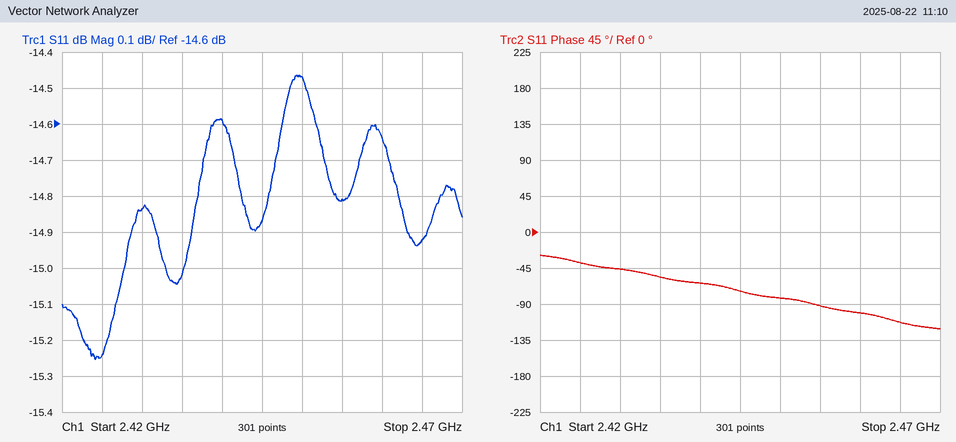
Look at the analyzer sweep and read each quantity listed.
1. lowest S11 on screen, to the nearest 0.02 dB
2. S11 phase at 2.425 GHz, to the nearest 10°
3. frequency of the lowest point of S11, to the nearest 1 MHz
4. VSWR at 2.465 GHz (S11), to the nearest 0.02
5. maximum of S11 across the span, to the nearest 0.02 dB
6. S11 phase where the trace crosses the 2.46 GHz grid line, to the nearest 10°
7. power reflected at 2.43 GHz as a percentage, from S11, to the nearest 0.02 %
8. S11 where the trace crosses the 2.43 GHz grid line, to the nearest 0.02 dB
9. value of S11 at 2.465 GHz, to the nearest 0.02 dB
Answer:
-15.26 dB
-40°
2.424 GHz
1.44
-14.46 dB
-100°
3.28 %
-14.84 dB
-14.92 dB
